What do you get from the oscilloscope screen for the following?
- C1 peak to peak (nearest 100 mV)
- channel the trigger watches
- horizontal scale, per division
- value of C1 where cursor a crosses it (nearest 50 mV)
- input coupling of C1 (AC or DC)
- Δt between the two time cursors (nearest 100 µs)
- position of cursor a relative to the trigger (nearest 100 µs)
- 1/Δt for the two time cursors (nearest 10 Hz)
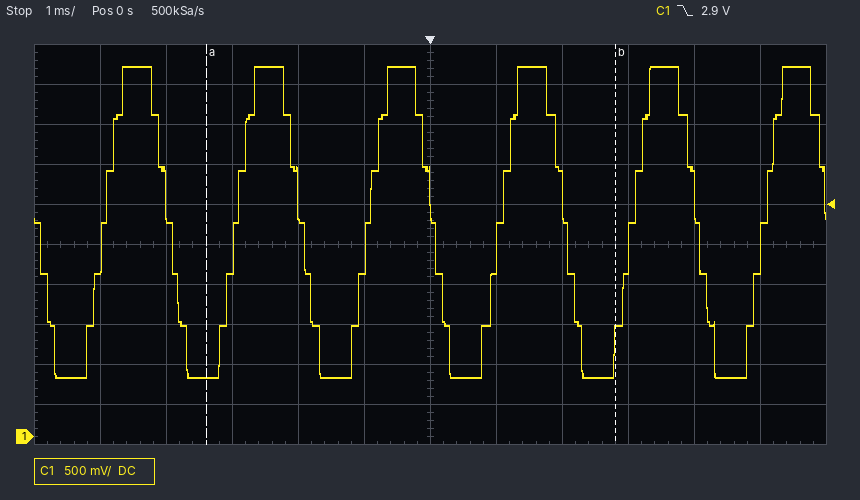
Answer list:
3.90 V
C1
1 ms
750 mV
DC
6.2 ms
-3.4 ms
160 Hz
